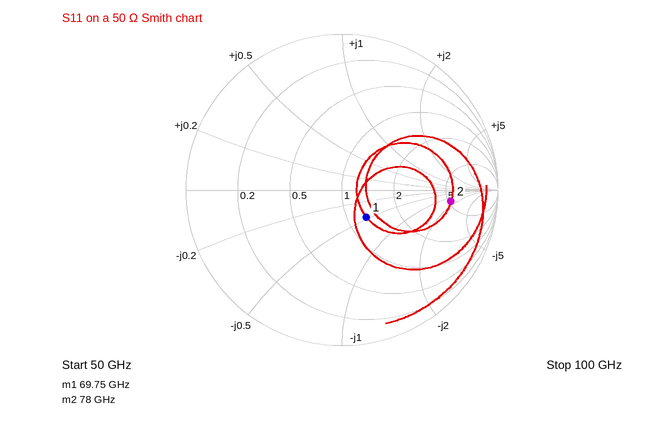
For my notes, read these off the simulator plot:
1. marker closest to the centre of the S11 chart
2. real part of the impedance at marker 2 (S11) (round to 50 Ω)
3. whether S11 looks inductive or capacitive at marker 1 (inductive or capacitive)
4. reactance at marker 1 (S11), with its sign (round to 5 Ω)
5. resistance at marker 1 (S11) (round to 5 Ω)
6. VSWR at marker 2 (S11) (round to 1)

marker 1
250 Ω
capacitive
-25 Ω
65 Ω
6
